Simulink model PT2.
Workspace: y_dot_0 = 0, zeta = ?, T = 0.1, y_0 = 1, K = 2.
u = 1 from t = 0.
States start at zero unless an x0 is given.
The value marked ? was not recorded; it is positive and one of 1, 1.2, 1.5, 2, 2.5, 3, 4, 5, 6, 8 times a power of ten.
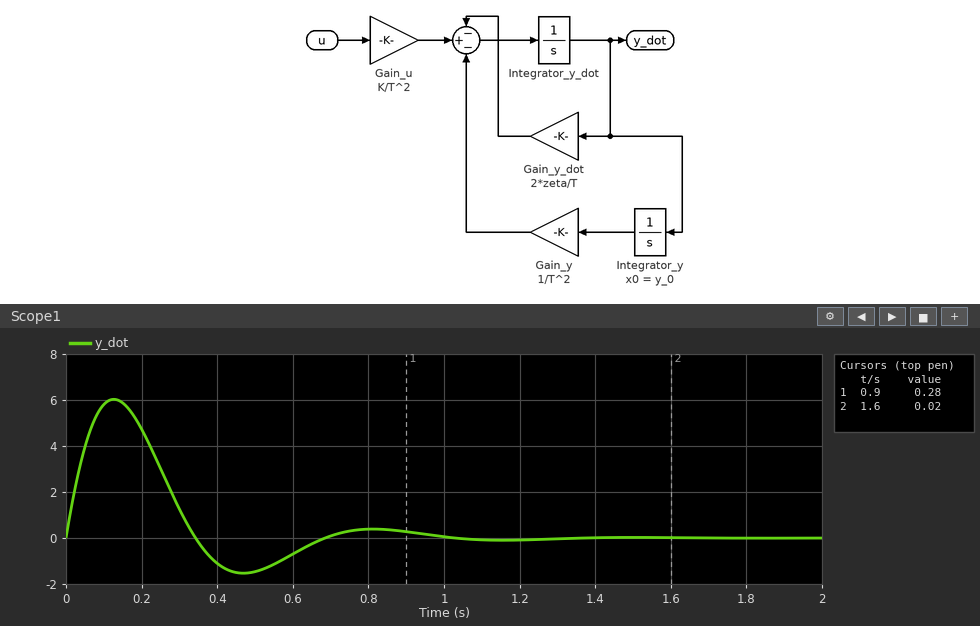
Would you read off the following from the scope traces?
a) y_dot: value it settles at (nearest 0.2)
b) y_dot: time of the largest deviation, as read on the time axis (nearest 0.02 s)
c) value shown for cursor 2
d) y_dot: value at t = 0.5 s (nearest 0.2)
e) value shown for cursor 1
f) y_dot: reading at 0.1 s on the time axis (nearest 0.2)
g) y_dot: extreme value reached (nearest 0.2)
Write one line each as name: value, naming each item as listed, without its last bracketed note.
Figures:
y_dot: value it settles at: 0.0
y_dot: time of the largest deviation, as read on the time axis: 0.12 s
value shown for cursor 2: 0.02
y_dot: value at t = 0.5 s: -1.4
value shown for cursor 1: 0.28
y_dot: reading at 0.1 s on the time axis: 5.8
y_dot: extreme value reached: 6.0
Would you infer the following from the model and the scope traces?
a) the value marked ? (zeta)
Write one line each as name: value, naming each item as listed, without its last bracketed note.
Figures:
the value marked ?: 0.4
